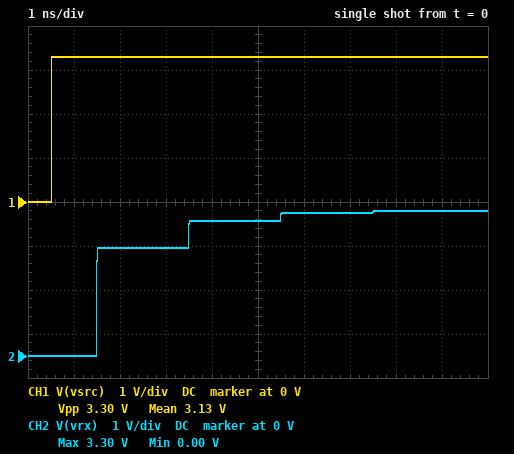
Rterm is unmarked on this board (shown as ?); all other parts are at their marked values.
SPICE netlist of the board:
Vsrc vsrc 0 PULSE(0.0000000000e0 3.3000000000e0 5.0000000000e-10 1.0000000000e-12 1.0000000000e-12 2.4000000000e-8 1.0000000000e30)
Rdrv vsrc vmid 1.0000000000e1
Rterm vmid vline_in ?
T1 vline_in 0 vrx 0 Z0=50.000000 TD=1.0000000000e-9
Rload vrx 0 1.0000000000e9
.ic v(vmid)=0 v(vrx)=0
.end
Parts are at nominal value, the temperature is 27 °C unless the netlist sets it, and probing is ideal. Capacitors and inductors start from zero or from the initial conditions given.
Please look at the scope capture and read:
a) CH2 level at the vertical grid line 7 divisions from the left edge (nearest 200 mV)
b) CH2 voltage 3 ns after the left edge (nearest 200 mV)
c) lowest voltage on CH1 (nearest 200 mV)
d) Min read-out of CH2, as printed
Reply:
3.2 V
2.4 V
0 V
0.00 V
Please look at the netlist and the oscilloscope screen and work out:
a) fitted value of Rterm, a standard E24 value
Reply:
75 Ω
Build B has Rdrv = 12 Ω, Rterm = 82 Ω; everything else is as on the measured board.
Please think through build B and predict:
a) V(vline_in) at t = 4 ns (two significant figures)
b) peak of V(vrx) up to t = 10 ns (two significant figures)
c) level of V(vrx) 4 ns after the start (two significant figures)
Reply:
2.6 V
3.3 V
3.0 V
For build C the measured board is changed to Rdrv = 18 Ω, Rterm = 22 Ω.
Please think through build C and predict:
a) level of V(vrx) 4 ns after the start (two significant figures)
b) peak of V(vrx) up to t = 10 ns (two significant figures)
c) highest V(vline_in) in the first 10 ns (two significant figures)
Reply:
3.3 V
3.7 V
3.5 V
